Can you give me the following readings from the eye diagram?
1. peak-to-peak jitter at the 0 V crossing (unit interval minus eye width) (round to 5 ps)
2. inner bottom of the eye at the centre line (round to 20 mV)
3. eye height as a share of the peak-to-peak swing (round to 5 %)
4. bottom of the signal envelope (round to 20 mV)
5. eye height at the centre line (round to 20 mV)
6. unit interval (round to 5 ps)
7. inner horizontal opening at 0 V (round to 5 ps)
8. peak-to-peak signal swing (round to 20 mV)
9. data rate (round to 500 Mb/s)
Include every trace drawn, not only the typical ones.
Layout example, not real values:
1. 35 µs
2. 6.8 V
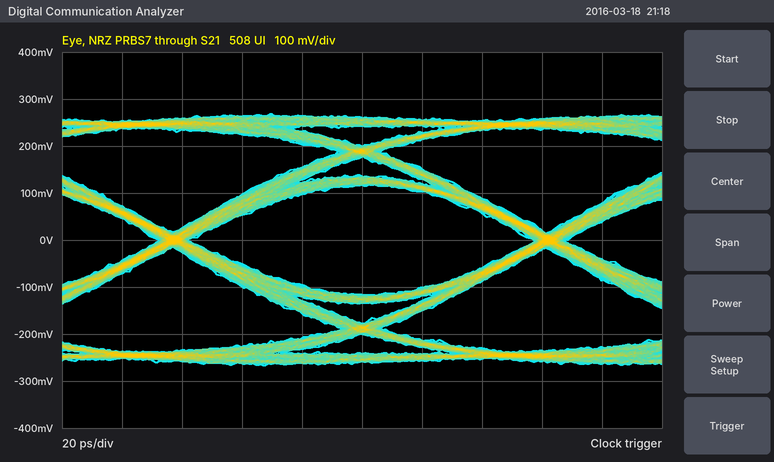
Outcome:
1. 10 ps
2. -120 mV
3. 45 %
4. -260 mV
5. 240 mV
6. 125 ps
7. 115 ps
8. 540 mV
9. 8.0 Gb/s
